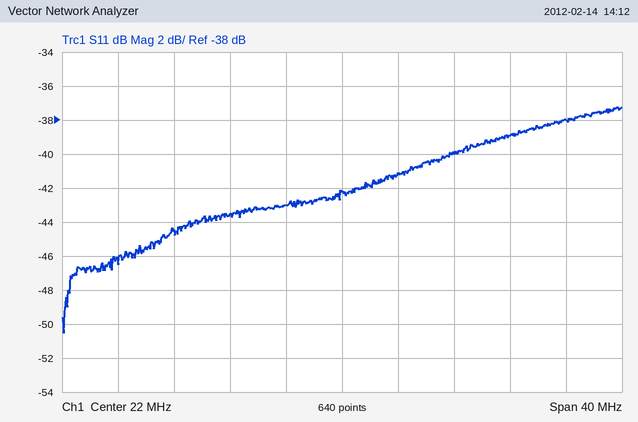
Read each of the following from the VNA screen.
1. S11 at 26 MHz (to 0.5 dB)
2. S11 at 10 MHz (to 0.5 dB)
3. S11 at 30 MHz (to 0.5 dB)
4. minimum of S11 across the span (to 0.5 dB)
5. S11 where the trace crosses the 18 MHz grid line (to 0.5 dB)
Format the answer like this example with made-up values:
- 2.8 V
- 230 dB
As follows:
- -41.0 dB
- -44.5 dB
- -40.0 dB
- -50.5 dB
- -43.0 dB
